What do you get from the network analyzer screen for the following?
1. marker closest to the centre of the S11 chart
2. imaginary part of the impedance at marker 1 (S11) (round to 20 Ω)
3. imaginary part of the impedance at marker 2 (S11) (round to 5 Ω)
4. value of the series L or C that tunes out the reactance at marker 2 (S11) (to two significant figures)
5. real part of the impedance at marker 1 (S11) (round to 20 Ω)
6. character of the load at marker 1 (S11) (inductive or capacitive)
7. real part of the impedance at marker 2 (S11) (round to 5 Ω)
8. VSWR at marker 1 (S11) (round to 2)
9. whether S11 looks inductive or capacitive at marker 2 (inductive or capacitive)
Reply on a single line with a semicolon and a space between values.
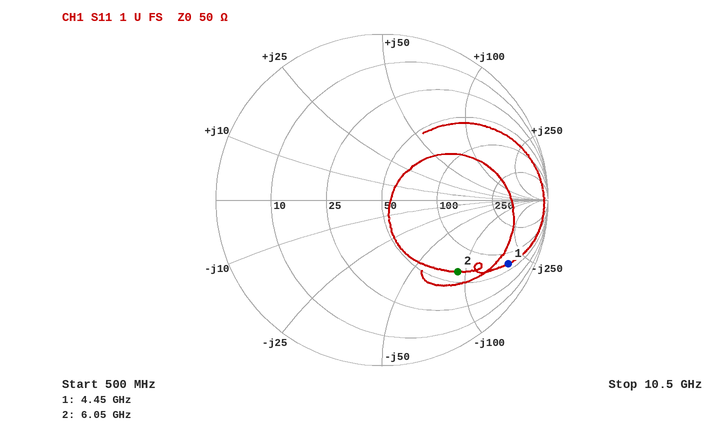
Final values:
marker 2; -180 Ω; -90 Ω; 2.4 nH; 60 Ω; capacitive; 65 Ω; 12; capacitive
